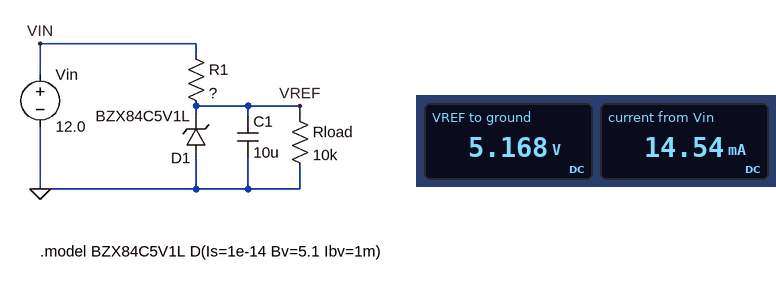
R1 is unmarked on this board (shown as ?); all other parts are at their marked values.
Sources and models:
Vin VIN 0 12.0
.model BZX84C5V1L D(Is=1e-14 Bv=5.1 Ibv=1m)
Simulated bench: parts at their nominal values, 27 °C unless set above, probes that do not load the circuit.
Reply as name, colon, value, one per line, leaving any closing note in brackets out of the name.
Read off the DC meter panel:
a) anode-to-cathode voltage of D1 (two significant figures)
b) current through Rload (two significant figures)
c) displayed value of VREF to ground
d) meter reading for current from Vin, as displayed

anode-to-cathode voltage of D1: -5.2 V
current through Rload: 520 µA
displayed value of VREF to ground: 5.168 V
meter reading for current from Vin, as displayed: 14.54 mA
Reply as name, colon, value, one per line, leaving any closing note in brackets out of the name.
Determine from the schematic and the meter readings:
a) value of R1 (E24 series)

value of R1: 470 Ω
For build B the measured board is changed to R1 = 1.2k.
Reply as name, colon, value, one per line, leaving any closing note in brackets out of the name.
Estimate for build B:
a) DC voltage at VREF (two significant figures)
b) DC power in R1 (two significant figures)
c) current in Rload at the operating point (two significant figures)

DC voltage at VREF: 5.1 V
DC power in R1: 39 mW
current in Rload at the operating point: 510 µA
